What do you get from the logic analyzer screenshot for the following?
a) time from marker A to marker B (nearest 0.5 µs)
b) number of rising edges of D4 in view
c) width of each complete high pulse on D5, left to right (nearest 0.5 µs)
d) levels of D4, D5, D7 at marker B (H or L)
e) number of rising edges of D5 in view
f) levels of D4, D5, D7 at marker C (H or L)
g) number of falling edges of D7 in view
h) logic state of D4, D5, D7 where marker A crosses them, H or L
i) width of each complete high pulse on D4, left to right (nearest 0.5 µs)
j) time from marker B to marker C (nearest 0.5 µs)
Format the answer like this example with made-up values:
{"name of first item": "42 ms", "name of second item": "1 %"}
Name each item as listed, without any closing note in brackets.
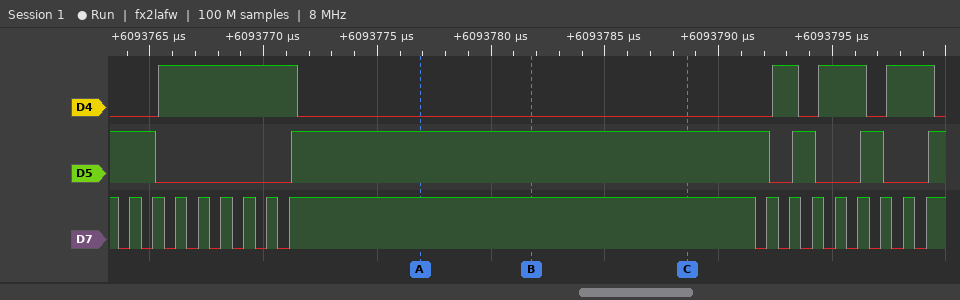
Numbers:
{"time from marker A to marker B": "5 µs", "number of rising edges of D4 in view": "4", "width of each complete high pulse on D5, left to right": "21 µs, 1 µs, 1 µs", "levels of D4, D5, D7 at marker B": "D4=L, D5=H, D7=H", "number of rising edges of D5 in view": "4", "levels of D4, D5, D7 at marker C": "D4=L, D5=H, D7=H", "number of falling edges of D7 in view": "16", "logic state of D4, D5, D7 where marker A crosses them, H or L": "D4=L, D5=H, D7=H", "width of each complete high pulse on D4, left to right": "6 µs, 1 µs, 2 µs, 2 µs", "time from marker B to marker C": "7 µs"}
